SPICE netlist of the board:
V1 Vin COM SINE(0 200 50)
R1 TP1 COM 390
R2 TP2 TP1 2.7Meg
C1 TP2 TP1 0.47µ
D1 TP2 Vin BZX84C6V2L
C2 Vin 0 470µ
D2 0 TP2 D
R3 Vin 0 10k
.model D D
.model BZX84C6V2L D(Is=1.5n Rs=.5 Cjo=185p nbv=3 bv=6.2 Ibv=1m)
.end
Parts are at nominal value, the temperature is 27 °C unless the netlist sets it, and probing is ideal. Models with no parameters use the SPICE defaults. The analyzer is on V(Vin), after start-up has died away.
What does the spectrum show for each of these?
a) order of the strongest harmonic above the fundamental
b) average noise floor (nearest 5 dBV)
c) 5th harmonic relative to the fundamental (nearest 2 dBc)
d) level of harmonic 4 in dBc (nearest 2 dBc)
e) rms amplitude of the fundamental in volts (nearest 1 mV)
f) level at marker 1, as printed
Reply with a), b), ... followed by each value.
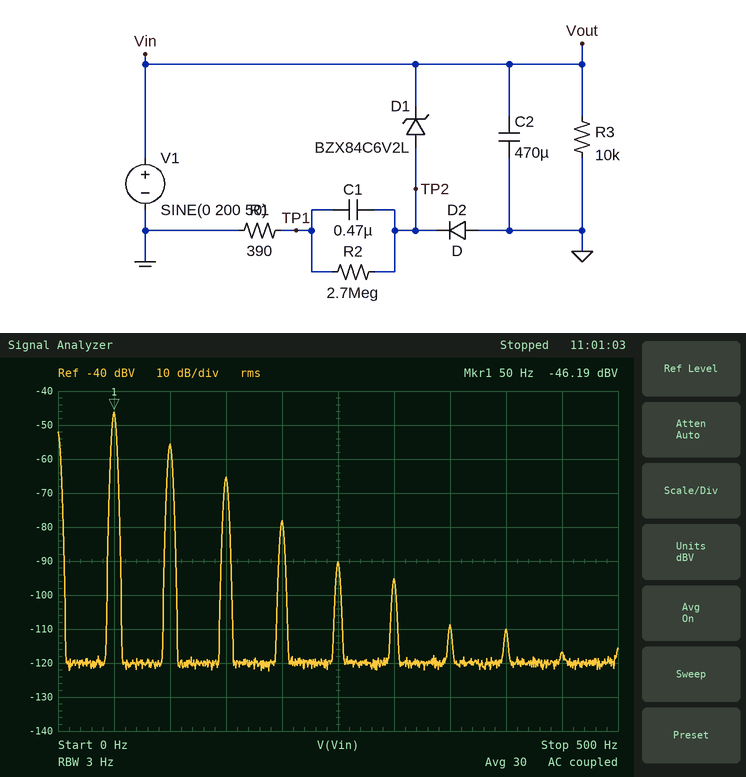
a) 2
b) -120 dBV
c) -44 dBc
d) -32 dBc
e) 5 mV
f) -46.19 dBV
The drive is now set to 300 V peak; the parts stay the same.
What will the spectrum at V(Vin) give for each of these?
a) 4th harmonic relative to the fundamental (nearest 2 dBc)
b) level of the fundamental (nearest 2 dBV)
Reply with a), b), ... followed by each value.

a) -30 dBc
b) -46 dBV
